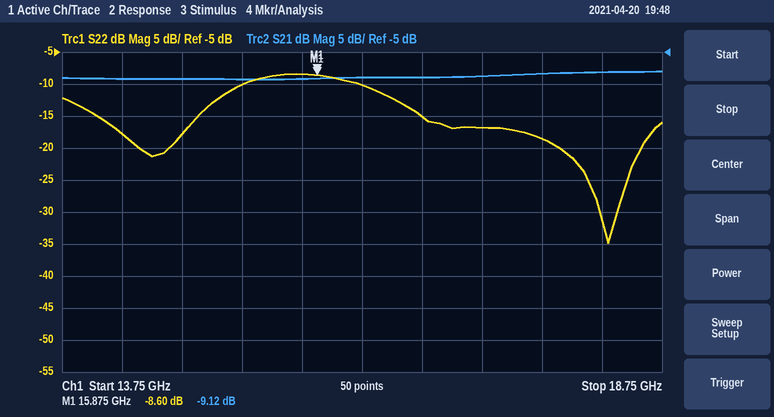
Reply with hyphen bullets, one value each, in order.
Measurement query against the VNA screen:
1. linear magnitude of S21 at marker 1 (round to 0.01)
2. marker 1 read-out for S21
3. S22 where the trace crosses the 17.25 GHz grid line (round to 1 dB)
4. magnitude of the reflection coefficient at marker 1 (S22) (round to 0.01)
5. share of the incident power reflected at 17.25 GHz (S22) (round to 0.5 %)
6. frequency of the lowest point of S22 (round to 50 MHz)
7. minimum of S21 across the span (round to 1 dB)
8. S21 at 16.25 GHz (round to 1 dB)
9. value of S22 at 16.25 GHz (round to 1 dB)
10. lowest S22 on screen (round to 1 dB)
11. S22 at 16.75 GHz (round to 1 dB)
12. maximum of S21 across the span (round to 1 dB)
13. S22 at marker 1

- 0.35
- -9.12 dB
- -17 dB
- 0.37
- 2.0 %
- 18.30 GHz
- -9 dB
- -9 dB
- -10 dB
- -35 dB
- -15 dB
- -8 dB
- -8.60 dB
